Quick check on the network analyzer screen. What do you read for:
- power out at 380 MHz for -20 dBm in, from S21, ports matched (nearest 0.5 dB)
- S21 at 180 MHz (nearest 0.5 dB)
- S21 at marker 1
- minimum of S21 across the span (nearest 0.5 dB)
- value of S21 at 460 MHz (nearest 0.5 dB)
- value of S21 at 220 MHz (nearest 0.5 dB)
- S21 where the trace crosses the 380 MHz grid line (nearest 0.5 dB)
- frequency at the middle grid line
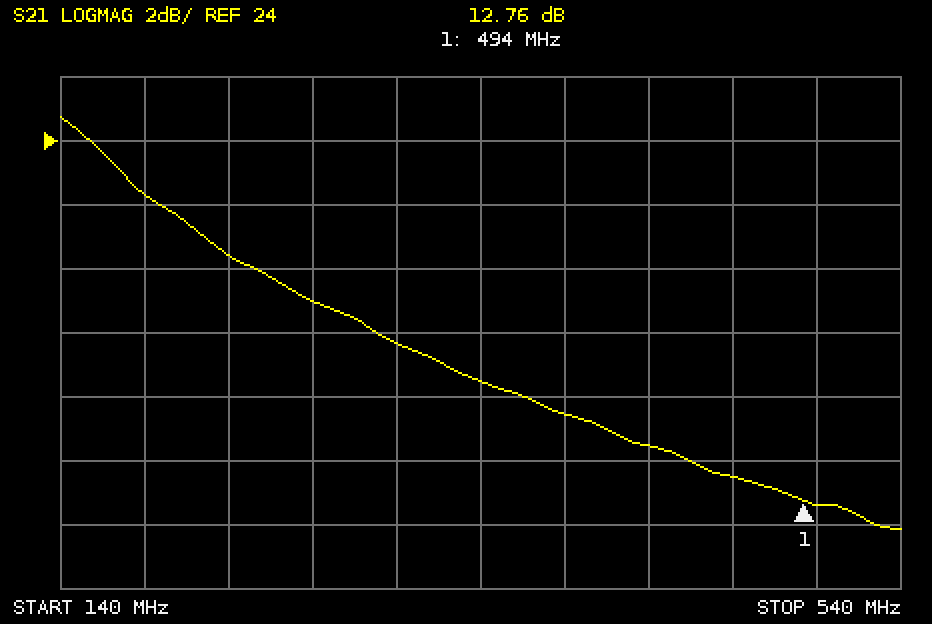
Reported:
-4.5 dBm
22.5 dB
12.76 dB
12.0 dB
13.5 dB
20.5 dB
15.5 dB
340 MHz
